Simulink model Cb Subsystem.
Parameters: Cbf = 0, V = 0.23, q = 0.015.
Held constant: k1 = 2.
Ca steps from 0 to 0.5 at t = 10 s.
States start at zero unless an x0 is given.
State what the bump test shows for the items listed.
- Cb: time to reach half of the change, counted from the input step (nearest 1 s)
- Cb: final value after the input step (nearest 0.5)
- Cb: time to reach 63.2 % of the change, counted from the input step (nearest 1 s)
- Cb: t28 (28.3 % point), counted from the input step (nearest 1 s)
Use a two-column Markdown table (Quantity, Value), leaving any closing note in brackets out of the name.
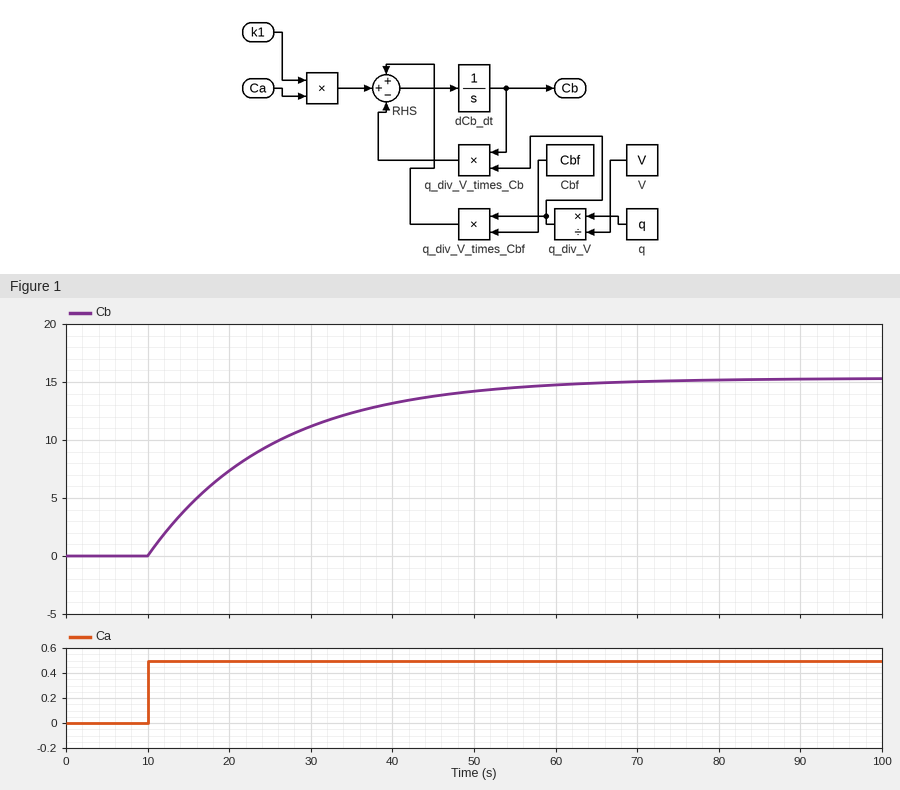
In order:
| Quantity | Value |
|---|---|
| Cb: time to reach half of the change, counted from the input step | 11 s |
| Cb: final value after the input step | 15.5 |
| Cb: time to reach 63.2 % of the change, counted from the input step | 15 s |
| Cb: t28 (28.3 % point), counted from the input step | 5 s |
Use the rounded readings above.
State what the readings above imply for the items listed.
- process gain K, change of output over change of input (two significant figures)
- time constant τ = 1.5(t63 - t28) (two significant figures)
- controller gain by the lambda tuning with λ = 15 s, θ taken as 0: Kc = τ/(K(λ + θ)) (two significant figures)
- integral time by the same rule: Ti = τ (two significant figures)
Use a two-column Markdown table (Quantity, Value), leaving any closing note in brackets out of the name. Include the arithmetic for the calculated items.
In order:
| Quantity | Value |
|---|---|
| process gain K, change of output over change of input | (15.5 - 0) / 0.5 = 31 |
| time constant τ = 1.5(t63 - t28) | 1.5 × (15 - 5) = 15 s |
| controller gain by the lambda tuning with λ = 15 s, θ taken as 0: Kc = τ/(K(λ + θ)) | 15 / (31 × (15 + 0)) = 0.032 |
| integral time by the same rule: Ti = τ | 15 s |
